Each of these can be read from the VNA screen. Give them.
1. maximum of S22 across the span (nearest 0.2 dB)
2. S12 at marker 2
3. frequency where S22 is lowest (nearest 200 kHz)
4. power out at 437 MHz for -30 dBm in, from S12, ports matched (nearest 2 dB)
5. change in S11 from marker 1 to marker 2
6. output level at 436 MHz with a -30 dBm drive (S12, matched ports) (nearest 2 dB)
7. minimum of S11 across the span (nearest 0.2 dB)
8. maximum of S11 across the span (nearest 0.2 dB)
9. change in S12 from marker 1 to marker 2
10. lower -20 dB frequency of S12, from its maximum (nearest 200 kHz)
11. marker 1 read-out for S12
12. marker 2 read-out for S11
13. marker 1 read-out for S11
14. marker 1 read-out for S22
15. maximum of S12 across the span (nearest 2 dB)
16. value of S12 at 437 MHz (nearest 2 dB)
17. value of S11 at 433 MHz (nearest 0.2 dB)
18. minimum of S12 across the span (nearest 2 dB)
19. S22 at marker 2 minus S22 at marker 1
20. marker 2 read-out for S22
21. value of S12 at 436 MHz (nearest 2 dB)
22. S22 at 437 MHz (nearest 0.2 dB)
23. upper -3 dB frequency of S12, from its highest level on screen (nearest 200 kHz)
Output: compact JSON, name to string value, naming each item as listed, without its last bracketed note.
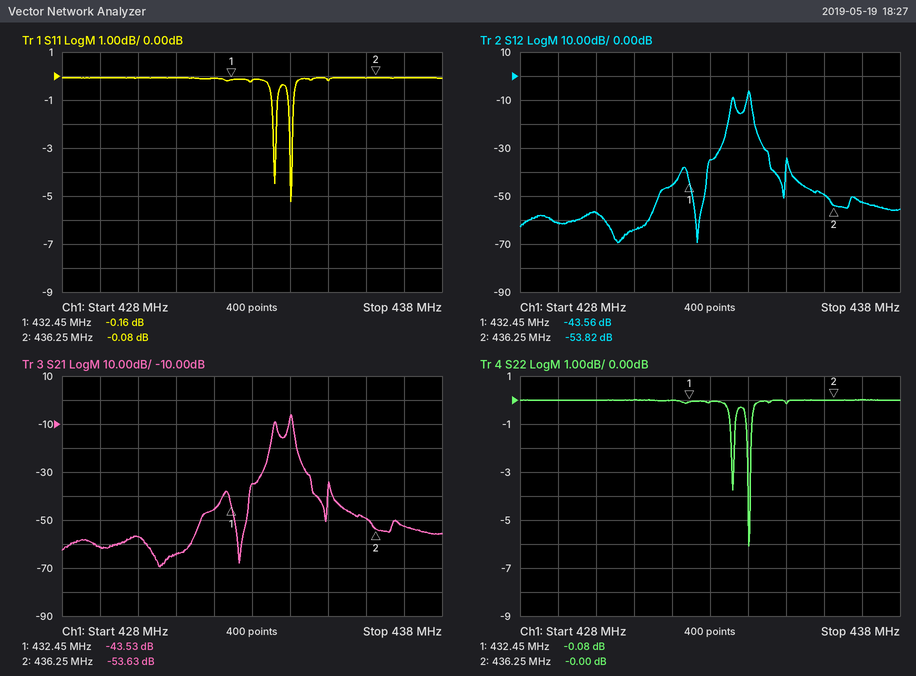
{"maximum of S22 across the span": "0.0 dB", "S12 at marker 2": "-53.82 dB", "frequency where S22 is lowest": "434.0 MHz", "power out at 437 MHz for -30 dBm in, from S12, ports matched": "-82 dBm", "change in S11 from marker 1 to marker 2": "0.08 dB", "output level at 436 MHz with a -30 dBm drive (S12, matched ports)": "-80 dBm", "minimum of S11 across the span": "-5.2 dB", "maximum of S11 across the span": "0.0 dB", "change in S12 from marker 1 to marker 2": "-10.26 dB", "lower -20 dB frequency of S12, from its maximum": "433.4 MHz", "marker 1 read-out for S12": "-43.56 dB", "marker 2 read-out for S11": "-0.08 dB", "marker 1 read-out for S11": "-0.16 dB", "marker 1 read-out for S22": "-0.08 dB", "maximum of S12 across the span": "-6 dB", "value of S12 at 437 MHz": "-52 dB", "value of S11 at 433 MHz": "-0.2 dB", "minimum of S12 across the span": "-70 dB", "S22 at marker 2 minus S22 at marker 1": "0.08 dB", "marker 2 read-out for S22": "-0.00 dB", "value of S12 at 436 MHz": "-50 dB", "S22 at 437 MHz": "0.0 dB", "upper -3 dB frequency of S12, from its highest level on screen": "434.0 MHz"}
